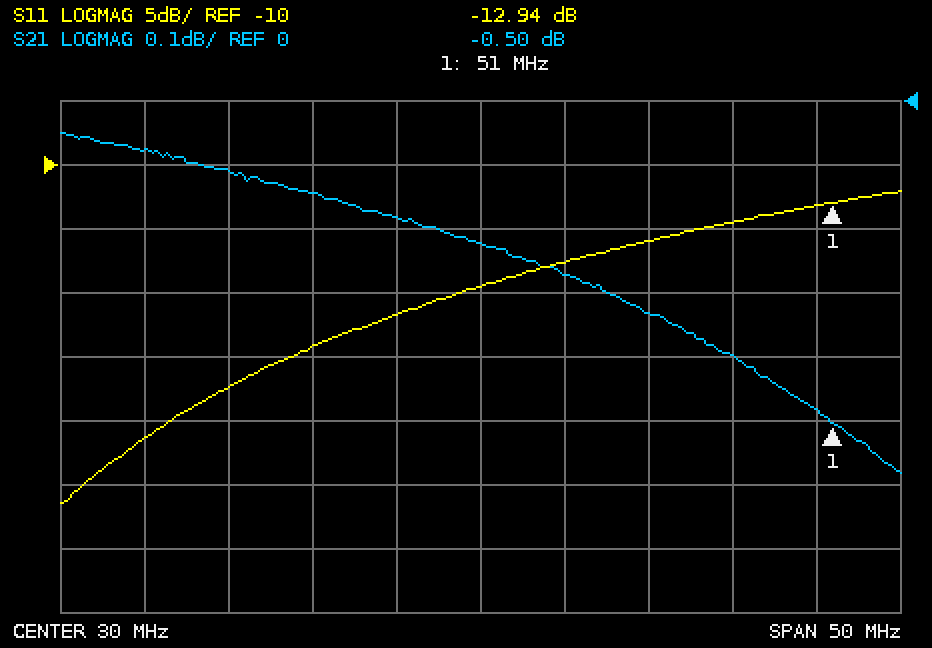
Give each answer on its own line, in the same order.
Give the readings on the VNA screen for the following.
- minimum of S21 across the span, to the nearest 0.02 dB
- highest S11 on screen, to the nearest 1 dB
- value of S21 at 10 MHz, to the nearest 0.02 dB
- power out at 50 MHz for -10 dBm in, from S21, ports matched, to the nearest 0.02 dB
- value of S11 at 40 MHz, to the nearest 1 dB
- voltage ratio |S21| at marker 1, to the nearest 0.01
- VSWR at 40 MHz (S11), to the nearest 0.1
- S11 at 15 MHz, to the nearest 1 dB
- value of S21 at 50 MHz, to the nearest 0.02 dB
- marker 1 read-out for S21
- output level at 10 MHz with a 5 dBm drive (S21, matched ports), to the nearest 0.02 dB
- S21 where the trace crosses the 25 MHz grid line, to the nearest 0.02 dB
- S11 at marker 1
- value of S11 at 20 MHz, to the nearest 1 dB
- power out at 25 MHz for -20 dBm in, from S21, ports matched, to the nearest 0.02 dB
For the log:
-0.58 dB
-12 dB
-0.08 dB
-10.48 dBm
-16 dB
0.94
1.4
-27 dB
-0.48 dB
-0.50 dB
4.92 dBm
-0.18 dB
-12.94 dB
-24 dB
-20.18 dBm
